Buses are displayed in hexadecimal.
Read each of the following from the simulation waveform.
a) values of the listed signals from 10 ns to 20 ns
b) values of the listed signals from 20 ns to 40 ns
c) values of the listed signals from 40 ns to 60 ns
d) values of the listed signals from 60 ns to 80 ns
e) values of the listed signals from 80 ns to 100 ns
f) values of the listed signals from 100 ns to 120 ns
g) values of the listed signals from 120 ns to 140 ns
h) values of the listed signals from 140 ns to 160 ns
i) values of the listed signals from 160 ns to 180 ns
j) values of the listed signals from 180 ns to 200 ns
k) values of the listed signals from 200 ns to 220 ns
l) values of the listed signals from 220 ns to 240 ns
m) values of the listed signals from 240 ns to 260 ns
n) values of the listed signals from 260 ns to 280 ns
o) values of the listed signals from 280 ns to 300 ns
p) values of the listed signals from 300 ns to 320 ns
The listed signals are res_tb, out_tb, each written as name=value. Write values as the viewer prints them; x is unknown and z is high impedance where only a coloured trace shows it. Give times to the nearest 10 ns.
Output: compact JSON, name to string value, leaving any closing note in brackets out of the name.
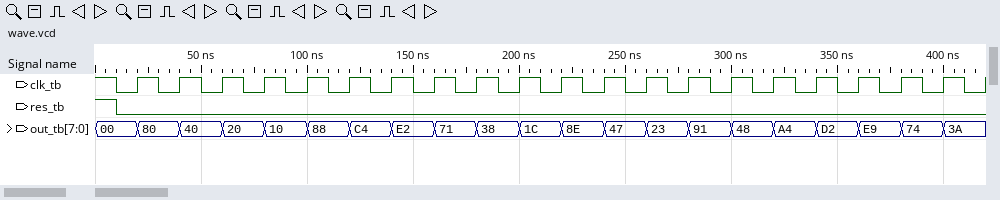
{"values of the listed signals from 10 ns to 20 ns": "res_tb=0, out_tb=00", "values of the listed signals from 20 ns to 40 ns": "res_tb=0, out_tb=80", "values of the listed signals from 40 ns to 60 ns": "res_tb=0, out_tb=40", "values of the listed signals from 60 ns to 80 ns": "res_tb=0, out_tb=20", "values of the listed signals from 80 ns to 100 ns": "res_tb=0, out_tb=10", "values of the listed signals from 100 ns to 120 ns": "res_tb=0, out_tb=88", "values of the listed signals from 120 ns to 140 ns": "res_tb=0, out_tb=C4", "values of the listed signals from 140 ns to 160 ns": "res_tb=0, out_tb=E2", "values of the listed signals from 160 ns to 180 ns": "res_tb=0, out_tb=71", "values of the listed signals from 180 ns to 200 ns": "res_tb=0, out_tb=38", "values of the listed signals from 200 ns to 220 ns": "res_tb=0, out_tb=1C", "values of the listed signals from 220 ns to 240 ns": "res_tb=0, out_tb=8E", "values of the listed signals from 240 ns to 260 ns": "res_tb=0, out_tb=47", "values of the listed signals from 260 ns to 280 ns": "res_tb=0, out_tb=23", "values of the listed signals from 280 ns to 300 ns": "res_tb=0, out_tb=91", "values of the listed signals from 300 ns to 320 ns": "res_tb=0, out_tb=48"}
